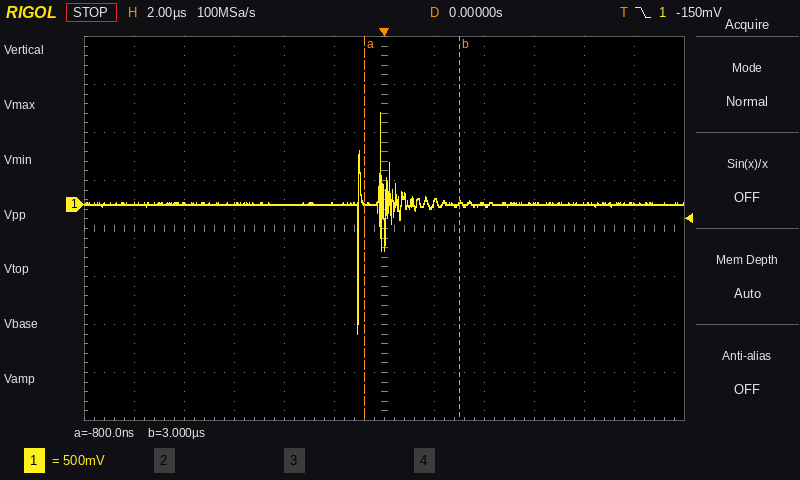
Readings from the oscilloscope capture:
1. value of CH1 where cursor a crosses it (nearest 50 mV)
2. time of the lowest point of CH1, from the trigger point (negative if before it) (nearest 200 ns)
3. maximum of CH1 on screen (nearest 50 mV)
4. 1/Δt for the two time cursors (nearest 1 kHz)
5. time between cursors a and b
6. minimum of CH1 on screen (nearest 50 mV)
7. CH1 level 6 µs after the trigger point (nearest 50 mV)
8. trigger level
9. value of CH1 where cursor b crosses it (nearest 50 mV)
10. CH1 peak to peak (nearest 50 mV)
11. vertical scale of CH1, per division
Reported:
50 mV
-1.0 µs
950 mV
263 kHz
3.8 µs
-1.35 V
0 mV
-150 mV
0 mV
2.30 V
500 mV
